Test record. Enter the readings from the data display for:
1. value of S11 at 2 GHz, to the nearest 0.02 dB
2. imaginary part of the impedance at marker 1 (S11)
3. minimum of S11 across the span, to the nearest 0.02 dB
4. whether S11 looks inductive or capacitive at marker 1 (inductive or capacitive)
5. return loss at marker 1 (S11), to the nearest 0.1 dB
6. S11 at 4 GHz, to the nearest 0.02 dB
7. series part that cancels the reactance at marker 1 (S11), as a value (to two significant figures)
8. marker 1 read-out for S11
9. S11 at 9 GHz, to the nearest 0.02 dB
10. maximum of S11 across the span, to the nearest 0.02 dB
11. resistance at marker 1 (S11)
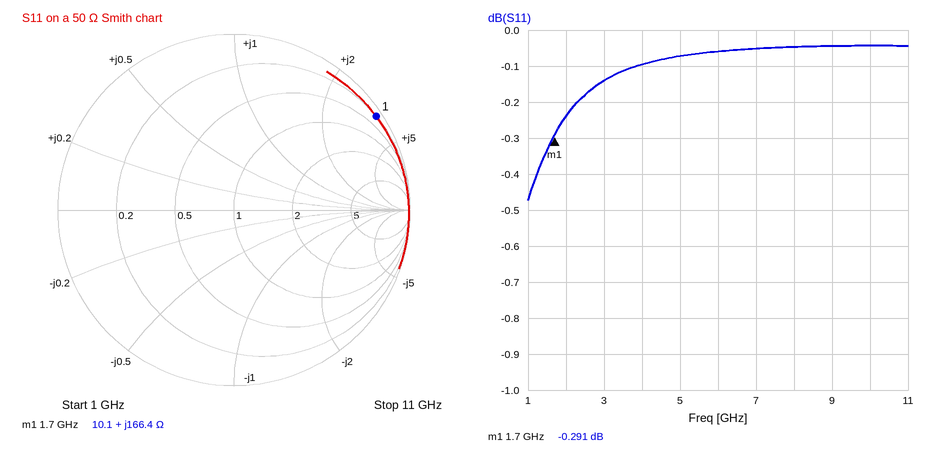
-0.24 dB
+166.4 Ω
-0.48 dB
inductive
0.3 dB
-0.10 dB
560 fF
-0.291 dB
-0.04 dB
-0.04 dB
10.1 Ω
